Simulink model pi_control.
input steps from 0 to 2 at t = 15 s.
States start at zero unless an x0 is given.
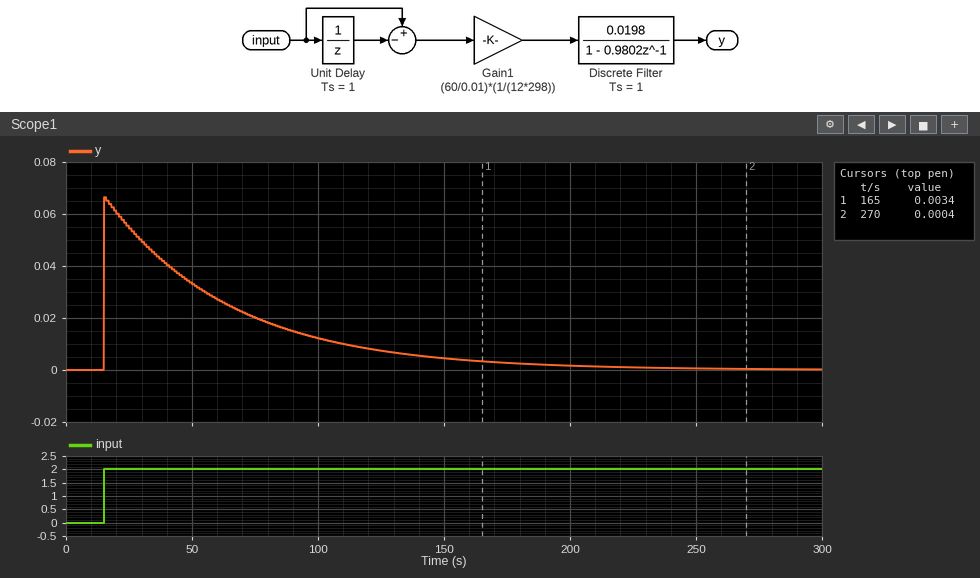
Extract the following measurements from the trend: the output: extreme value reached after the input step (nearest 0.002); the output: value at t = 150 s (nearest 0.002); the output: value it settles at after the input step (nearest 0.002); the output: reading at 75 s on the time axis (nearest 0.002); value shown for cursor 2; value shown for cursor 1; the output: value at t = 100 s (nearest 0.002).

0.066
0.004
0.000
0.020
0.0004
0.0034
0.012
